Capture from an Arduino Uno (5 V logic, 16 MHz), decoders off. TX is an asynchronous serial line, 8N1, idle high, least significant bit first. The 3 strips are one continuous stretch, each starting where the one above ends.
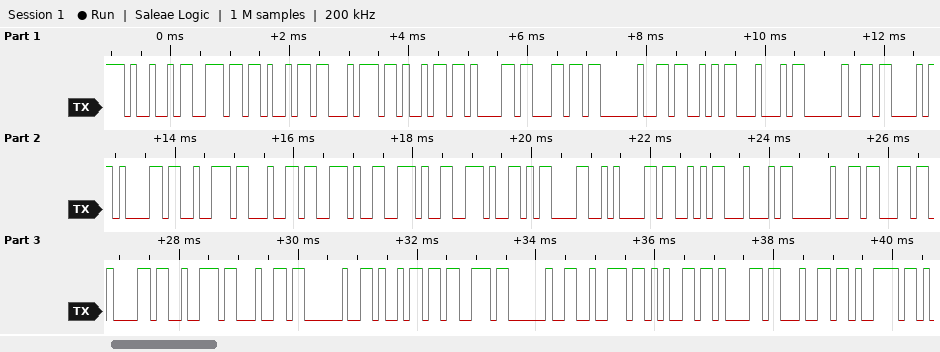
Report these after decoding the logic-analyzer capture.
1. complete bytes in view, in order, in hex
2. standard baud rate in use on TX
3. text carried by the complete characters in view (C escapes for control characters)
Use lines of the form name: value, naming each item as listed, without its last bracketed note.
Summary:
complete bytes in view, in order, in hex: 0x49 0x6E 0x69 0x74 0x69 0x61 0x6C 0x20 0x53 0x44 0x20 0x43 0x61 0x72 0x64 0x2E 0x2E 0x2E 0x0D 0x0A 0x53 0x44 0x20 0x63 0x61 0x72 0x64 0x20 0x69 0x73 0x20 0x72 0x65 0x61 0x64 0x79
standard baud rate in use on TX: 9600 baud
text carried by the complete characters in view: "Initial SD Card...\r\nSD card is ready"
